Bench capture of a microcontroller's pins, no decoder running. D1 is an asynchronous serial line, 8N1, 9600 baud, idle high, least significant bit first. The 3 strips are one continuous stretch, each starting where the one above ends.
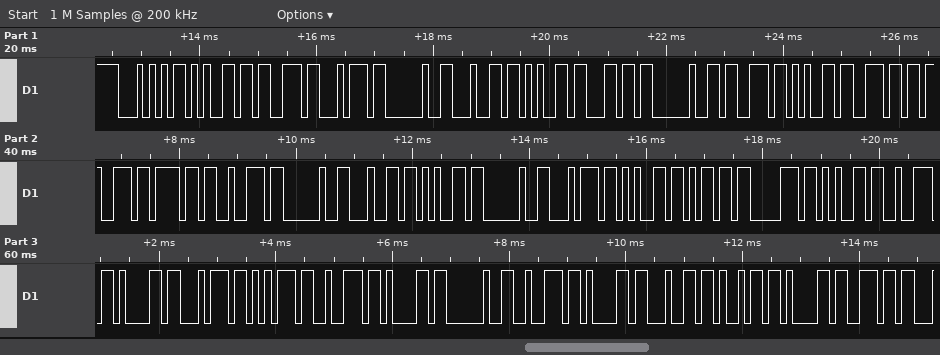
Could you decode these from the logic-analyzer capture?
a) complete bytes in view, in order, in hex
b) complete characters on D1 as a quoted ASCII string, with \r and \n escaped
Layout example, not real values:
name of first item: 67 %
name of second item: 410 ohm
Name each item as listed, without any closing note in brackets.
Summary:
complete bytes in view, in order, in hex: 54 65 73 74 20 64 65 6C 20 73 65 6E 73 6F 72 20 64 65 20 74 65 6D 70 65 72 61 74 75 72 61 20 72 61 64 69 61 6E
complete characters on D1 as a quoted ASCII string, with \r and \n escaped: "Test del sensor de temperatura radian"
